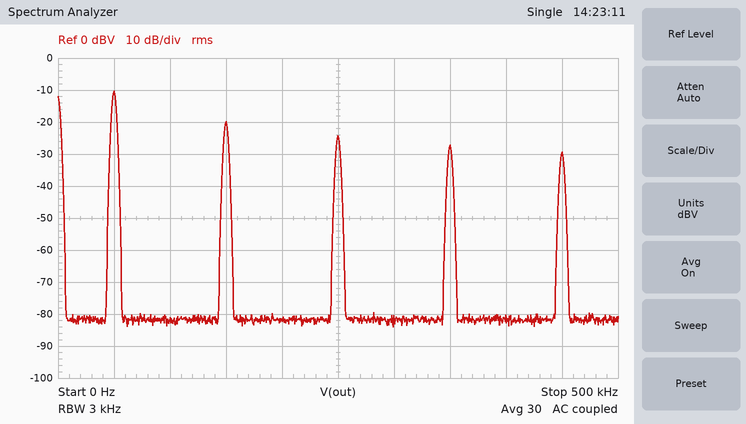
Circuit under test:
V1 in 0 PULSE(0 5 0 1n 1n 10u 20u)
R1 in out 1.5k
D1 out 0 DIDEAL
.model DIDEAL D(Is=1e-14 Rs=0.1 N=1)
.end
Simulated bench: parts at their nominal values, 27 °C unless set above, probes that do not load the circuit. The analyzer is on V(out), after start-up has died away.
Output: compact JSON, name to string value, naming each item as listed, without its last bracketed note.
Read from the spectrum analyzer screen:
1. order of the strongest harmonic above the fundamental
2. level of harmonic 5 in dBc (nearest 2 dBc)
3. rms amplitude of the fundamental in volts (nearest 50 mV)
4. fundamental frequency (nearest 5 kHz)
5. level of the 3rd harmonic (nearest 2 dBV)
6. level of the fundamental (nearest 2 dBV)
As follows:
{"order of the strongest harmonic above the fundamental": "3", "level of harmonic 5 in dBc": "-14 dBc", "rms amplitude of the fundamental in volts": "300 mV", "fundamental frequency": "50 kHz", "level of the 3rd harmonic": "-20 dBV", "level of the fundamental": "-10 dBV"}
